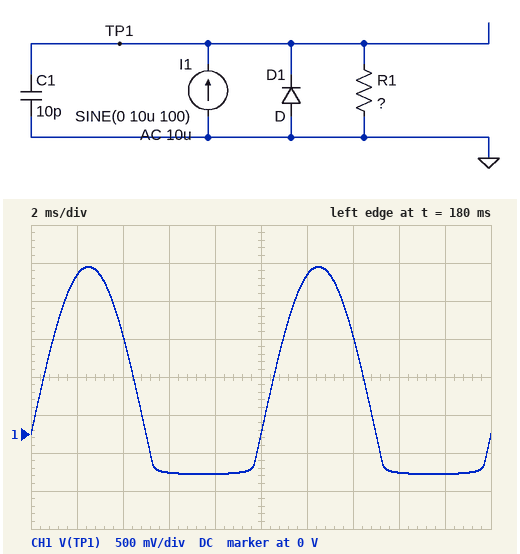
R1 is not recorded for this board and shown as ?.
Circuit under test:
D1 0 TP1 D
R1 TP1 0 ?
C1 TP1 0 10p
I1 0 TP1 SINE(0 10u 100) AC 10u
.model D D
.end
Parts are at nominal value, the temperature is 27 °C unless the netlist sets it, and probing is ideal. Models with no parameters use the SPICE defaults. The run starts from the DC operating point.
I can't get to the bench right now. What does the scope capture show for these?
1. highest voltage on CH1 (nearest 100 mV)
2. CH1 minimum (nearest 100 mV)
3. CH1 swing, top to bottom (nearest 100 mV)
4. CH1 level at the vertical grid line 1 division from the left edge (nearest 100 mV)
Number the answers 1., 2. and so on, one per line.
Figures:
1. 2.2 V
2. -500 mV
3. 2.7 V
4. 2.1 V
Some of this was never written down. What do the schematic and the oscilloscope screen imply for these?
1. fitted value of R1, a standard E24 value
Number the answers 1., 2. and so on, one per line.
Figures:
1. 220 kΩ
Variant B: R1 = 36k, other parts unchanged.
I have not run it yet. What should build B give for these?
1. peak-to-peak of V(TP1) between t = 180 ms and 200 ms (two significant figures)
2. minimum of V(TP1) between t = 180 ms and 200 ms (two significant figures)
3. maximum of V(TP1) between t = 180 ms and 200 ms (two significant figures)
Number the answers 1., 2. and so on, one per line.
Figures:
1. 720 mV
2. -360 mV
3. 360 mV
